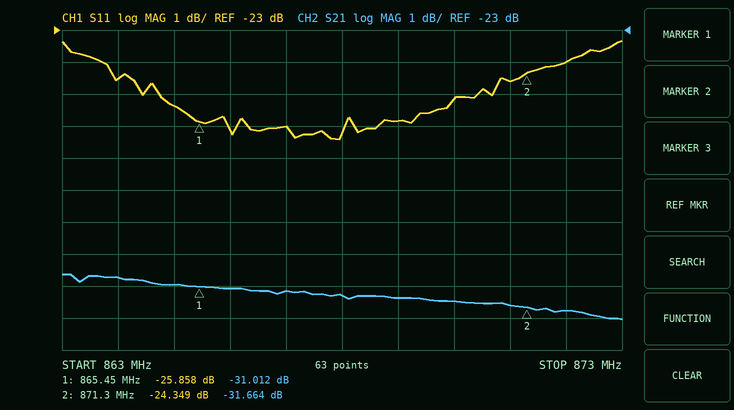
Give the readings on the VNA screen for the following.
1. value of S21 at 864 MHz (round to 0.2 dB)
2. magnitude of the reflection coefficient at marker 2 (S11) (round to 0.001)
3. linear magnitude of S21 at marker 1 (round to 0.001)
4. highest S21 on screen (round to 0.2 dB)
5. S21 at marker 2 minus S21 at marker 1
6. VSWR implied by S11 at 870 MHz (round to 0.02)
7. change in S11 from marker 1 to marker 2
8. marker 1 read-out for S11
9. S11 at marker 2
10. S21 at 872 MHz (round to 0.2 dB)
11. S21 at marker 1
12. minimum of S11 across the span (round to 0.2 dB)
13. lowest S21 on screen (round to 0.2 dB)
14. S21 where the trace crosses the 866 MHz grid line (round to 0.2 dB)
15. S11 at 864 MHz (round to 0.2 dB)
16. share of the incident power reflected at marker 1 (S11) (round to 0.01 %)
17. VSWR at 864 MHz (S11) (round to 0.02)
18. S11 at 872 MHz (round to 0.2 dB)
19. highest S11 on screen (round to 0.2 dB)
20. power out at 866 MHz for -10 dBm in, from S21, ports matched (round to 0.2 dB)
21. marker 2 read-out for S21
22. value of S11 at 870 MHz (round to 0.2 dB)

-30.8 dB
0.061
0.028
-30.6 dB
-0.652 dB
1.12
1.509 dB
-25.858 dB
-24.349 dB
-31.8 dB
-31.012 dB
-26.4 dB
-32.0 dB
-31.0 dB
-24.6 dB
0.26 %
1.12
-24.0 dB
-23.4 dB
-41.0 dBm
-31.664 dB
-25.2 dB
